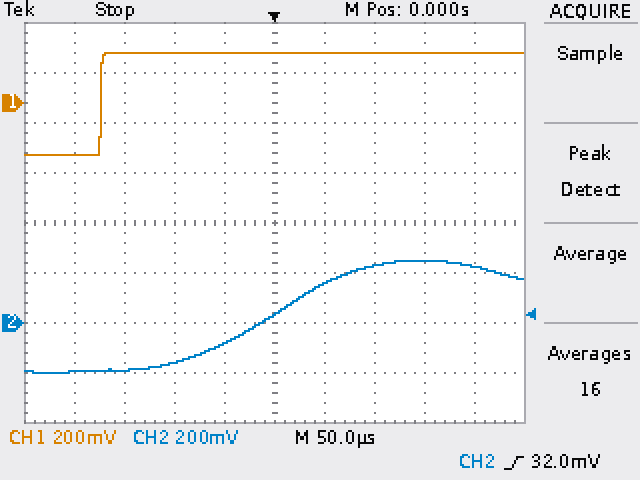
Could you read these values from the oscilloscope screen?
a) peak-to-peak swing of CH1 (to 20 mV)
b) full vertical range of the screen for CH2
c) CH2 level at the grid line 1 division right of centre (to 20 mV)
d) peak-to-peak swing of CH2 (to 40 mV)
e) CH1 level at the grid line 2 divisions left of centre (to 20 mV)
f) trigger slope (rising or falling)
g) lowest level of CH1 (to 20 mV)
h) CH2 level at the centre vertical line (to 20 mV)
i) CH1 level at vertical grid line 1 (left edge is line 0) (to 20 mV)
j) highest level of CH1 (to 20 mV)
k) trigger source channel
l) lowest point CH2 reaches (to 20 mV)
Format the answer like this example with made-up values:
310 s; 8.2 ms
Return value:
400 mV; 1.6 V; 160 mV; 440 mV; 200 mV; rising; -200 mV; 40 mV; -200 mV; 200 mV; CH2; -200 mV
